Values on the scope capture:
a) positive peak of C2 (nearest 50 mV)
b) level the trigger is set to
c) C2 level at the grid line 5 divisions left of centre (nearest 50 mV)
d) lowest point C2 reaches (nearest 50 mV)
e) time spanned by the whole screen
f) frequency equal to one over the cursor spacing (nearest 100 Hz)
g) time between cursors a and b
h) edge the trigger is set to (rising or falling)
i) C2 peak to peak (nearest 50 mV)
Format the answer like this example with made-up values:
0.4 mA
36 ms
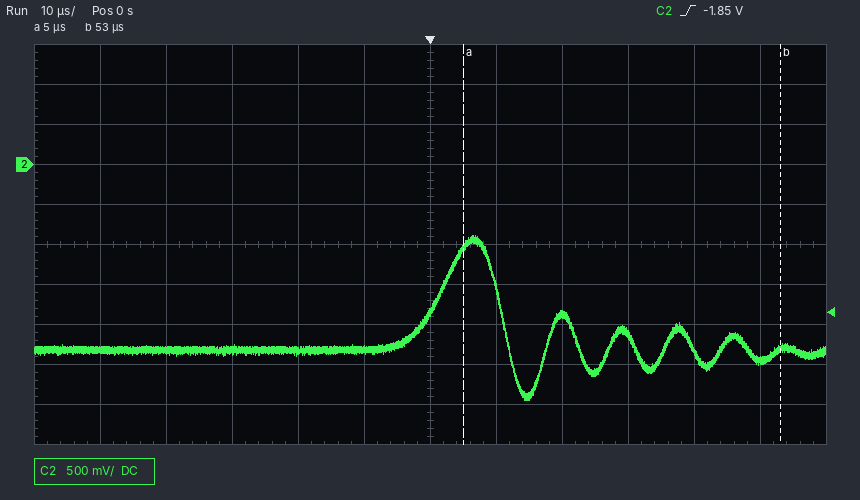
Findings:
-900 mV
-1.85 V
-2.30 V
-2.95 V
120 µs
20.8 kHz
48 µs
rising
2.05 V
